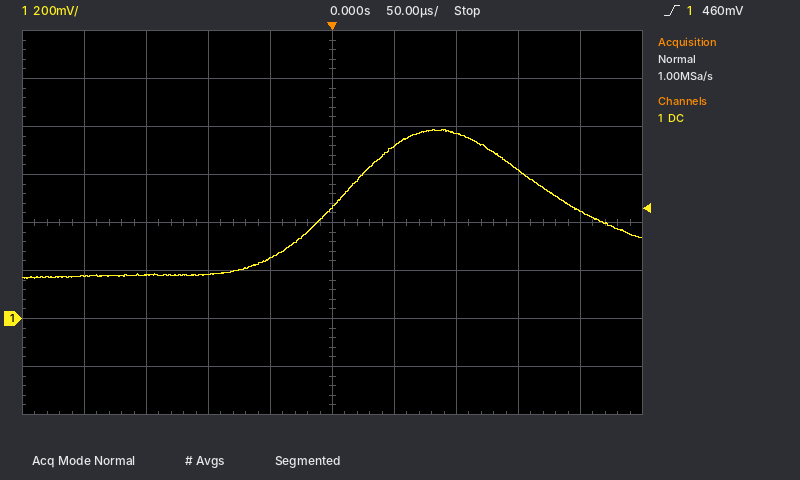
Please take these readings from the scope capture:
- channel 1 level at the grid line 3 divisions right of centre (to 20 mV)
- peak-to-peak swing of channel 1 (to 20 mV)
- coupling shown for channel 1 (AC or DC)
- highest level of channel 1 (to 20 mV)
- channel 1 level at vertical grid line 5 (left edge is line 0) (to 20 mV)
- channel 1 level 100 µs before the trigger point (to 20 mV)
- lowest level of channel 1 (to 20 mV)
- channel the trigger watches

620 mV
620 mV
DC
780 mV
460 mV
180 mV
160 mV
channel 1
